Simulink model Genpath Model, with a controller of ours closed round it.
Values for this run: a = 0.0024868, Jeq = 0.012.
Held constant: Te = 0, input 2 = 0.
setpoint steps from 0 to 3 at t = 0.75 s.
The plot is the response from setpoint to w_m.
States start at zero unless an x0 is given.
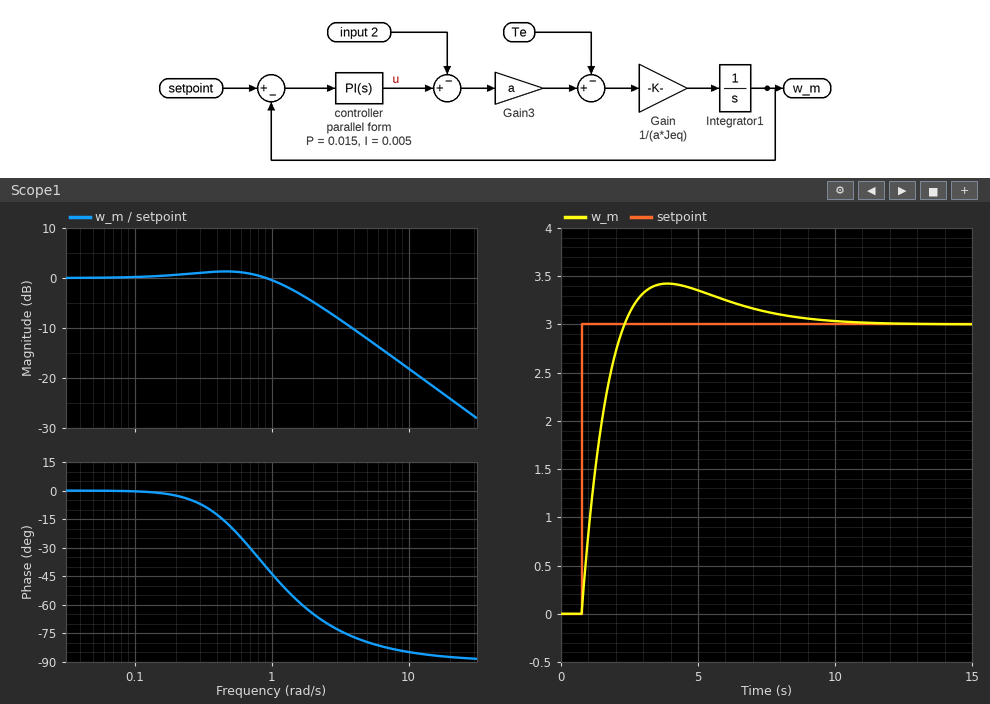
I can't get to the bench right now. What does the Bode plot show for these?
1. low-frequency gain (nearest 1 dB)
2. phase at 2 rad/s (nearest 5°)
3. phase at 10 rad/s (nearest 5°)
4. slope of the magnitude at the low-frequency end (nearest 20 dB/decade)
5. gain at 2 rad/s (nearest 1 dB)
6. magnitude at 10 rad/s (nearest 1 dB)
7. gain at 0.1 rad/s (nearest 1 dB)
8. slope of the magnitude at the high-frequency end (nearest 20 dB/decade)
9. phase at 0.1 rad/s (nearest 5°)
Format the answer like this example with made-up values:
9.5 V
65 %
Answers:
0 dB
-65°
-85°
0 dB/decade
-5 dB
-18 dB
0 dB
-20 dB/decade
0°
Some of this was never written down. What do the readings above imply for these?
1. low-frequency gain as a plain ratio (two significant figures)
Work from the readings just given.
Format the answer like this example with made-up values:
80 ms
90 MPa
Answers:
1.0
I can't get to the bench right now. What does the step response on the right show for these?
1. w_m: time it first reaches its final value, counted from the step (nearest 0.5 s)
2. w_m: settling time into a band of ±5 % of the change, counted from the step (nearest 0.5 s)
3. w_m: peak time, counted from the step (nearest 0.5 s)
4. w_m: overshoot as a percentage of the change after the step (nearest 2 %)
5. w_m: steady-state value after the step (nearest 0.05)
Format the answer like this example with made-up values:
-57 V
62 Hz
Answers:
1.5 s
6.5 s
3.0 s
14 %
3.00
